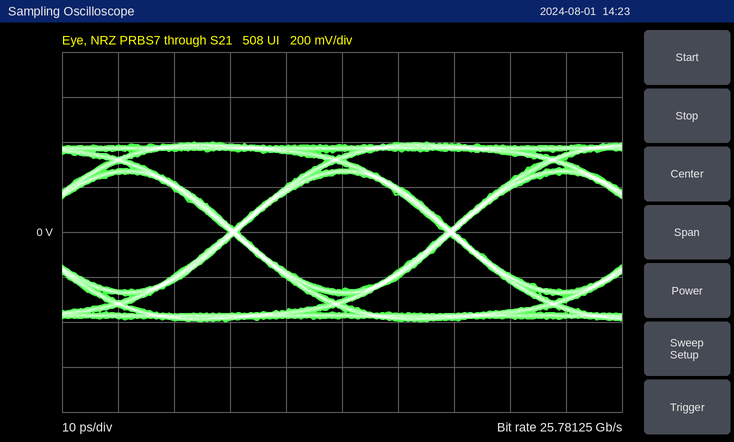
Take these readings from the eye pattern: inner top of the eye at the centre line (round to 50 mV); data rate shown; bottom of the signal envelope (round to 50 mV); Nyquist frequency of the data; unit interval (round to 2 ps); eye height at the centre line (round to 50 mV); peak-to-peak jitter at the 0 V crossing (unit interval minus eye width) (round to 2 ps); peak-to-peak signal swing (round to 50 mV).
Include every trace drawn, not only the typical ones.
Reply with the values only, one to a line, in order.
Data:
250 mV
25.78125 Gb/s
-400 mV
12.89062 GHz
38 ps
500 mV
2 ps
800 mV
